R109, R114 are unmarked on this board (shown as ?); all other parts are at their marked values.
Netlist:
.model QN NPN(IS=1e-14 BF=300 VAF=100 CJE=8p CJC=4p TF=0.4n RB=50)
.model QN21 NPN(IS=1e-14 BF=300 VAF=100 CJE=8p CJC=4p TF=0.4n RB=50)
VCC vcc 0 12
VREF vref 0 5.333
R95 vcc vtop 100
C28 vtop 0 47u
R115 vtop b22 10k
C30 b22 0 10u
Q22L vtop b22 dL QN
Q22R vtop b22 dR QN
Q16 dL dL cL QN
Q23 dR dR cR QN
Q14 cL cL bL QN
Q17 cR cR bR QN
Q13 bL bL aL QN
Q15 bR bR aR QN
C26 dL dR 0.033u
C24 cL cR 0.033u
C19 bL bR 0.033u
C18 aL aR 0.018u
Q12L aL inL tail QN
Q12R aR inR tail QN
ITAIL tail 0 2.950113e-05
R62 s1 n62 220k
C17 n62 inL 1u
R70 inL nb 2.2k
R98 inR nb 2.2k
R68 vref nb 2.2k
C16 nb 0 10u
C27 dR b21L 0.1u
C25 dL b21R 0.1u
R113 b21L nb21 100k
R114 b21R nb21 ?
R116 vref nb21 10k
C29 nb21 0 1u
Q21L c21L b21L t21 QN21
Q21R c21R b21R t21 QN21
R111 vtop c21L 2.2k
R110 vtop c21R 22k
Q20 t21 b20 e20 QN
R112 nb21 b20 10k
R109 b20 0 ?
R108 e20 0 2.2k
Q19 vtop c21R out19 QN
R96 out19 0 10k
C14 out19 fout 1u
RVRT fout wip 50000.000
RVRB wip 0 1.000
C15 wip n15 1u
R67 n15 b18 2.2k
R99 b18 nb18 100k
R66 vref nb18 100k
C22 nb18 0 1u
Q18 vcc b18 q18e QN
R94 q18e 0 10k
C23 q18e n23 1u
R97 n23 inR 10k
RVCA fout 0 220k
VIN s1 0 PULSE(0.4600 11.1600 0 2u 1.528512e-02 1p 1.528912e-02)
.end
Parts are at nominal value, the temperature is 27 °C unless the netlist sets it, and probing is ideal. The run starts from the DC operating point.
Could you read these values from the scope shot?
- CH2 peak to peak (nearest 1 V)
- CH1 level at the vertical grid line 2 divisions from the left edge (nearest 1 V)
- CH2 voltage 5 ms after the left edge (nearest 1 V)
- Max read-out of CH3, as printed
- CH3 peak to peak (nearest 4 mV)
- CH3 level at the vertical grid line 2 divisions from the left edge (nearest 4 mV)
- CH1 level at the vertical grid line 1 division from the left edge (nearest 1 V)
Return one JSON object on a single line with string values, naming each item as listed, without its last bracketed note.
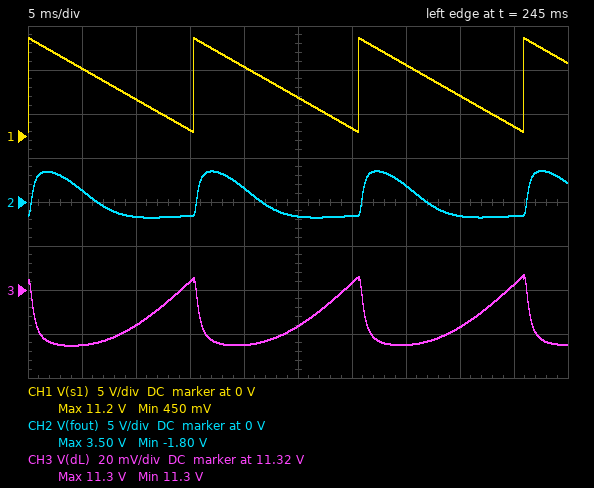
{"CH2 peak to peak": "5 V", "CH1 level at the vertical grid line 2 divisions from the left edge": "4 V", "CH2 voltage 5 ms after the left edge": "1 V", "Max read-out of CH3, as printed": "11.3 V", "CH3 peak to peak": "32 mV", "CH3 level at the vertical grid line 2 divisions from the left edge": "11.304 V", "CH1 level at the vertical grid line 1 division from the left edge": "8 V"}
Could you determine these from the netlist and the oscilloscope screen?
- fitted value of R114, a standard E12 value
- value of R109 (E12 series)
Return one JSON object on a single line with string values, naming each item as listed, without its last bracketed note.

{"fitted value of R114, a standard E12 value": "270 kΩ", "value of R109": "18 kΩ"}
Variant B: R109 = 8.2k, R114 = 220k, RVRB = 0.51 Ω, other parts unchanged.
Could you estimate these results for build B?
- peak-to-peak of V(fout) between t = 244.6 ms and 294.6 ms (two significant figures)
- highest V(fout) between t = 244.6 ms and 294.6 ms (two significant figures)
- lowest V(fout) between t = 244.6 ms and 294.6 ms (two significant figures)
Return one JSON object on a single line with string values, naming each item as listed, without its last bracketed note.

{"peak-to-peak of V(fout) between t = 244.6 ms and 294.6 ms": "3.5 V", "highest V(fout) between t = 244.6 ms and 294.6 ms": "2.1 V", "lowest V(fout) between t = 244.6 ms and 294.6 ms": "-1.4 V"}
